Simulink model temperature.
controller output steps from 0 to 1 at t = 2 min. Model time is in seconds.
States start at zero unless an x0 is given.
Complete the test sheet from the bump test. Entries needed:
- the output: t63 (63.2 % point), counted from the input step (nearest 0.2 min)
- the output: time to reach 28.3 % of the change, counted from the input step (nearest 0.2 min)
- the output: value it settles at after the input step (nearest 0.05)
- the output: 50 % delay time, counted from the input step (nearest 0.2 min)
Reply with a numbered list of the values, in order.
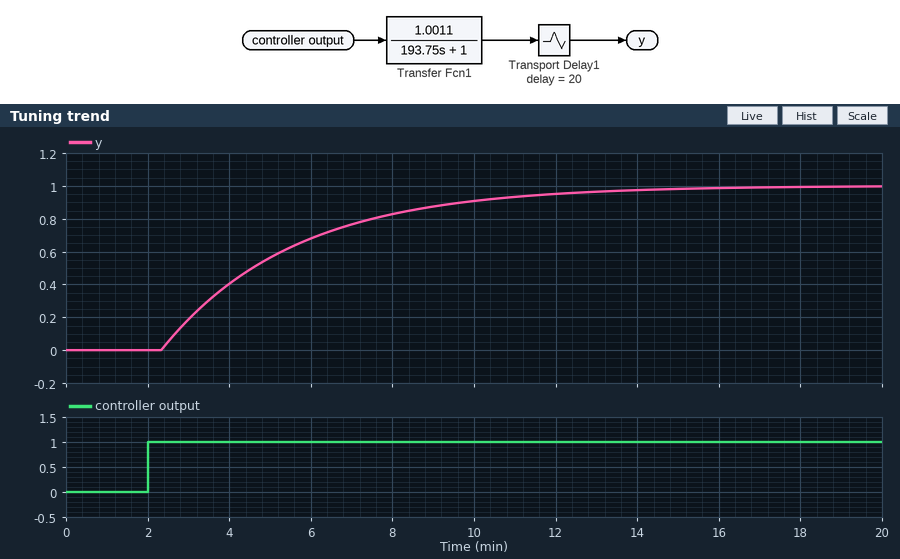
1. 3.6 min
2. 1.4 min
3. 1.00
4. 2.6 min
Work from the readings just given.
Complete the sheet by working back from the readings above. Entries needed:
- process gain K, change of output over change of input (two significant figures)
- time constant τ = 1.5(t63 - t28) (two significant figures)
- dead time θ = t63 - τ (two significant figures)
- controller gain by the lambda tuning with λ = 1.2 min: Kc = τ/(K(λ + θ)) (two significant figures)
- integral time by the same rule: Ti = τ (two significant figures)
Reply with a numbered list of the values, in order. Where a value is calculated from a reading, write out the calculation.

1. (1 - 0) / 1 = 1.0
2. 1.5 × (3.6 - 1.4) = 3.3 min
3. 3.6 - 3.3 = 0.30 min
4. 3.3 / (1 × (1.2 + 0.3)) = 2.2
5. 3.3 min
